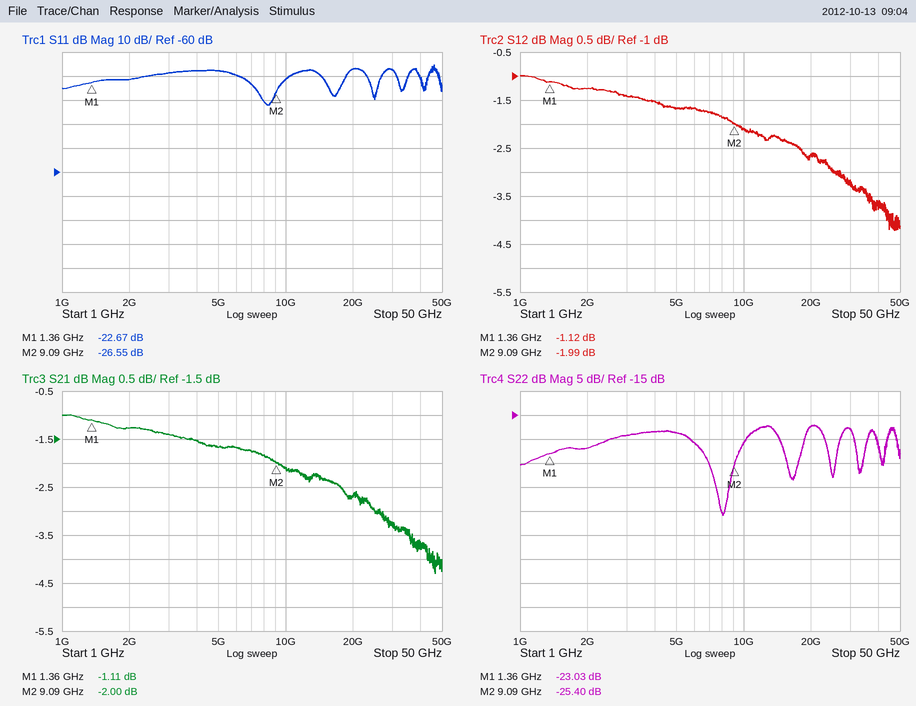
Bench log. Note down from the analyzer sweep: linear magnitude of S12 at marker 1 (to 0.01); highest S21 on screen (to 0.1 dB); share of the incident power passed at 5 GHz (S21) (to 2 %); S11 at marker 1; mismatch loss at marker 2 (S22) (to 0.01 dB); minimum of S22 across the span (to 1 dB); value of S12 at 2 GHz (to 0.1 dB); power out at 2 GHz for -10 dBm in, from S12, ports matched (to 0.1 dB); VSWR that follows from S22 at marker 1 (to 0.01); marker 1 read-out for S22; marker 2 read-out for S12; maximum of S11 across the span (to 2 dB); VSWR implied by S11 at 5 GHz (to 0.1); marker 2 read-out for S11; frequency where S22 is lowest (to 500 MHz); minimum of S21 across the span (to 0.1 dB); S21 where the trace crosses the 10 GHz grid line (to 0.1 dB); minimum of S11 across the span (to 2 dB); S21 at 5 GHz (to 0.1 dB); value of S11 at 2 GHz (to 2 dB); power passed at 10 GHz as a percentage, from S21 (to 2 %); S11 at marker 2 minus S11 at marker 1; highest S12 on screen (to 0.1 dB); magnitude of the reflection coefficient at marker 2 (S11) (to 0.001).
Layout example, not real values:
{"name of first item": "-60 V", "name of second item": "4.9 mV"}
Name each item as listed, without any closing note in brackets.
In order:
{"linear magnitude of S12 at marker 1": "0.88", "highest S21 on screen": "-1.0 dB", "share of the incident power passed at 5 GHz (S21)": "68 %", "S11 at marker 1": "-22.67 dB", "mismatch loss at marker 2 (S22)": "0.01 dB", "minimum of S22 across the span": "-36 dB", "value of S12 at 2 GHz": "-1.3 dB", "power out at 2 GHz for -10 dBm in, from S12, ports matched": "-11.3 dBm", "VSWR that follows from S22 at marker 1": "1.15", "marker 1 read-out for S22": "-23.03 dB", "marker 2 read-out for S12": "-1.99 dB", "maximum of S11 across the span": "-16 dB", "VSWR implied by S11 at 5 GHz": "1.3", "marker 2 read-out for S11": "-26.55 dB", "frequency where S22 is lowest": "8.0 GHz", "minimum of S21 across the span": "-4.3 dB", "S21 where the trace crosses the 10 GHz grid line": "-2.1 dB", "minimum of S11 across the span": "-32 dB", "S21 at 5 GHz": "-1.7 dB", "value of S11 at 2 GHz": "-22 dB", "power passed at 10 GHz as a percentage, from S21": "62 %", "S11 at marker 2 minus S11 at marker 1": "-3.88 dB", "highest S12 on screen": "-1.0 dB", "magnitude of the reflection coefficient at marker 2 (S11)": "0.047"}
